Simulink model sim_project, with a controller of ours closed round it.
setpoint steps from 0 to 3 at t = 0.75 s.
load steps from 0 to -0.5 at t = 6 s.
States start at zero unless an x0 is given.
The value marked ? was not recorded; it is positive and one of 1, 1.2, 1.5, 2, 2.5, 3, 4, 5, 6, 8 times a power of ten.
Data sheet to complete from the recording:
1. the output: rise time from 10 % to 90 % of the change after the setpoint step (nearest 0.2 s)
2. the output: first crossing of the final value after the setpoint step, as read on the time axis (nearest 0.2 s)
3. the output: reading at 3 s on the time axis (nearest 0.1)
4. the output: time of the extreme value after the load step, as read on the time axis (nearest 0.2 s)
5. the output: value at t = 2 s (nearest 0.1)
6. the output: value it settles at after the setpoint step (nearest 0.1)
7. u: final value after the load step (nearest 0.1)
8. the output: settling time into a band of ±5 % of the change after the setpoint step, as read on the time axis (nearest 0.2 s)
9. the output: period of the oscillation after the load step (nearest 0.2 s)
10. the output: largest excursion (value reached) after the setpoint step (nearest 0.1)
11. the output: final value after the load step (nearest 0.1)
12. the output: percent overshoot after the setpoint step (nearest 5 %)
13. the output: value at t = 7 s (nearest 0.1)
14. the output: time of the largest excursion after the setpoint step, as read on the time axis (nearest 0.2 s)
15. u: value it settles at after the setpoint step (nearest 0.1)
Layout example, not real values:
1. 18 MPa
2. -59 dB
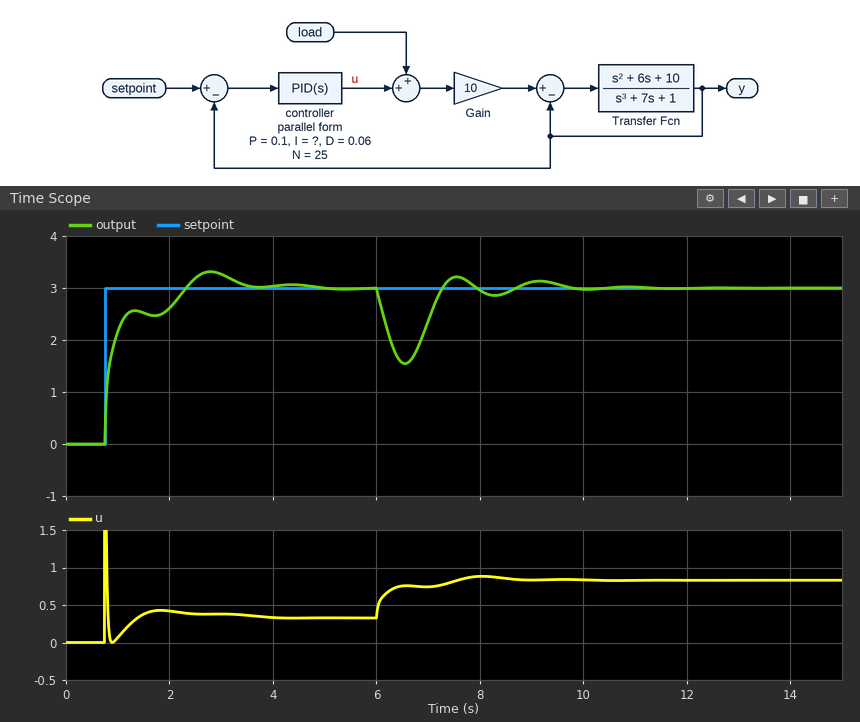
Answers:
1. 1.4 s
2. 2.4 s
3. 3.3
4. 6.6 s
5. 2.6
6. 3.0
7. 0.8
8. 3.2 s
9. 1.8 s
10. 3.3
11. 3.0
12. 10 %
13. 2.4
14. 2.8 s
15. 0.3
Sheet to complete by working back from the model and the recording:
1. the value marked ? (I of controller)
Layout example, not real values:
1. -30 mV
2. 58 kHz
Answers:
1. 0.5
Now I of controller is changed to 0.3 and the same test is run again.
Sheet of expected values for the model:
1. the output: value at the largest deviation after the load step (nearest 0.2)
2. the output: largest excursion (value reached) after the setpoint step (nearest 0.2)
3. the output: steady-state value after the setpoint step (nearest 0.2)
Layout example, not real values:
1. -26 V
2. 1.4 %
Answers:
1. 1.4
2. 3.2
3. 3.0
